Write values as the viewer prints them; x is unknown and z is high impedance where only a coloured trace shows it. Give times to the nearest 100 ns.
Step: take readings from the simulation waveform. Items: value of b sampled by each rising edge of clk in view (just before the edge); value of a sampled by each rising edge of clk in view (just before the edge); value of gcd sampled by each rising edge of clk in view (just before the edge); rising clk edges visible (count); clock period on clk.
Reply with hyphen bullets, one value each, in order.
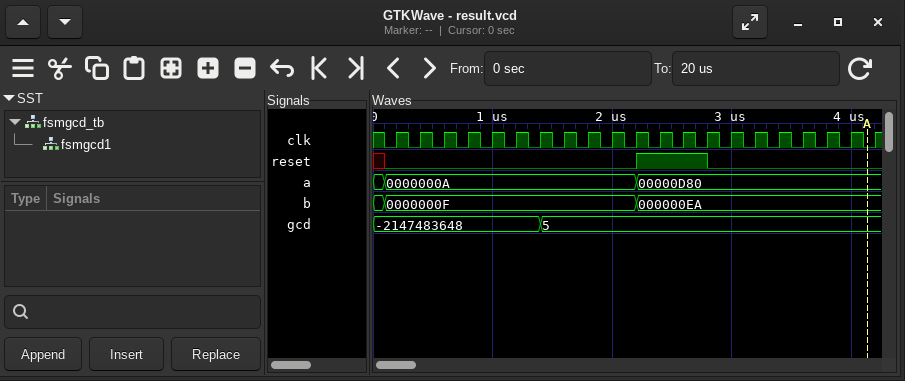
- 0000000F, 0000000F, 0000000F, 0000000F, 0000000F, 0000000F, 0000000F, 0000000F, 0000000F, 0000000F, 0000000F, 000000EA, 000000EA, 000000EA, 000000EA, 000000EA, 000000EA, 000000EA, 000000EA, 000000EA, 000000EA
- 0000000A, 0000000A, 0000000A, 0000000A, 0000000A, 0000000A, 0000000A, 0000000A, 0000000A, 0000000A, 0000000A, 00000D80, 00000D80, 00000D80, 00000D80, 00000D80, 00000D80, 00000D80, 00000D80, 00000D80, 00000D80
- -2147483648, -2147483648, -2147483648, -2147483648, -2147483648, -2147483648, -2147483648, 5, 5, 5, 5, 5, 5, 5, 5, 5, 5, 5, 5, 5, 5
- 21
- 200 ns
